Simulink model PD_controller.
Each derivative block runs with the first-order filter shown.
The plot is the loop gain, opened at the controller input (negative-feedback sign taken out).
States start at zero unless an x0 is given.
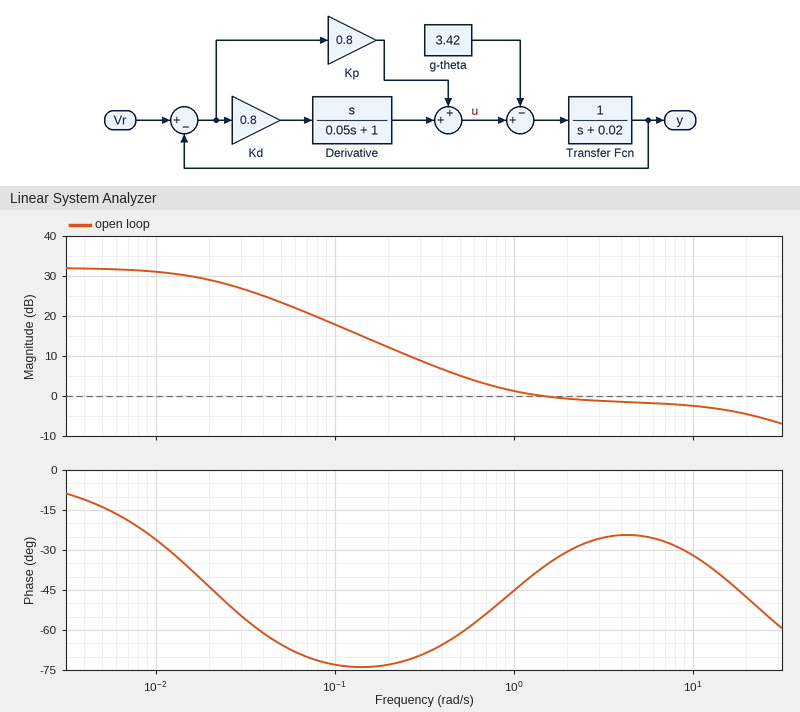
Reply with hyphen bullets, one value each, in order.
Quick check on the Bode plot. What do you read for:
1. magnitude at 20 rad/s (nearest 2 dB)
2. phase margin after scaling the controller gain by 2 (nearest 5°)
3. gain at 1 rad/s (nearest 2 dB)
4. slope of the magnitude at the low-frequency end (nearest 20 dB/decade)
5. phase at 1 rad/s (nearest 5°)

- -4 dB
- 125°
- 2 dB
- 0 dB/decade
- -45°
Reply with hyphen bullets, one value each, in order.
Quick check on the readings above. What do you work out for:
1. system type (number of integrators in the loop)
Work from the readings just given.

- 0
